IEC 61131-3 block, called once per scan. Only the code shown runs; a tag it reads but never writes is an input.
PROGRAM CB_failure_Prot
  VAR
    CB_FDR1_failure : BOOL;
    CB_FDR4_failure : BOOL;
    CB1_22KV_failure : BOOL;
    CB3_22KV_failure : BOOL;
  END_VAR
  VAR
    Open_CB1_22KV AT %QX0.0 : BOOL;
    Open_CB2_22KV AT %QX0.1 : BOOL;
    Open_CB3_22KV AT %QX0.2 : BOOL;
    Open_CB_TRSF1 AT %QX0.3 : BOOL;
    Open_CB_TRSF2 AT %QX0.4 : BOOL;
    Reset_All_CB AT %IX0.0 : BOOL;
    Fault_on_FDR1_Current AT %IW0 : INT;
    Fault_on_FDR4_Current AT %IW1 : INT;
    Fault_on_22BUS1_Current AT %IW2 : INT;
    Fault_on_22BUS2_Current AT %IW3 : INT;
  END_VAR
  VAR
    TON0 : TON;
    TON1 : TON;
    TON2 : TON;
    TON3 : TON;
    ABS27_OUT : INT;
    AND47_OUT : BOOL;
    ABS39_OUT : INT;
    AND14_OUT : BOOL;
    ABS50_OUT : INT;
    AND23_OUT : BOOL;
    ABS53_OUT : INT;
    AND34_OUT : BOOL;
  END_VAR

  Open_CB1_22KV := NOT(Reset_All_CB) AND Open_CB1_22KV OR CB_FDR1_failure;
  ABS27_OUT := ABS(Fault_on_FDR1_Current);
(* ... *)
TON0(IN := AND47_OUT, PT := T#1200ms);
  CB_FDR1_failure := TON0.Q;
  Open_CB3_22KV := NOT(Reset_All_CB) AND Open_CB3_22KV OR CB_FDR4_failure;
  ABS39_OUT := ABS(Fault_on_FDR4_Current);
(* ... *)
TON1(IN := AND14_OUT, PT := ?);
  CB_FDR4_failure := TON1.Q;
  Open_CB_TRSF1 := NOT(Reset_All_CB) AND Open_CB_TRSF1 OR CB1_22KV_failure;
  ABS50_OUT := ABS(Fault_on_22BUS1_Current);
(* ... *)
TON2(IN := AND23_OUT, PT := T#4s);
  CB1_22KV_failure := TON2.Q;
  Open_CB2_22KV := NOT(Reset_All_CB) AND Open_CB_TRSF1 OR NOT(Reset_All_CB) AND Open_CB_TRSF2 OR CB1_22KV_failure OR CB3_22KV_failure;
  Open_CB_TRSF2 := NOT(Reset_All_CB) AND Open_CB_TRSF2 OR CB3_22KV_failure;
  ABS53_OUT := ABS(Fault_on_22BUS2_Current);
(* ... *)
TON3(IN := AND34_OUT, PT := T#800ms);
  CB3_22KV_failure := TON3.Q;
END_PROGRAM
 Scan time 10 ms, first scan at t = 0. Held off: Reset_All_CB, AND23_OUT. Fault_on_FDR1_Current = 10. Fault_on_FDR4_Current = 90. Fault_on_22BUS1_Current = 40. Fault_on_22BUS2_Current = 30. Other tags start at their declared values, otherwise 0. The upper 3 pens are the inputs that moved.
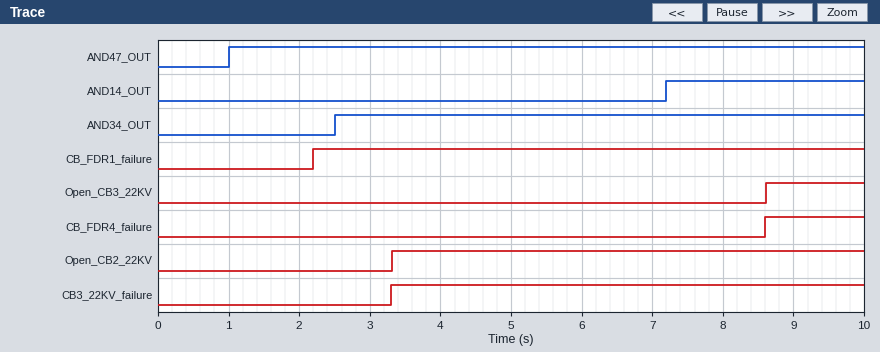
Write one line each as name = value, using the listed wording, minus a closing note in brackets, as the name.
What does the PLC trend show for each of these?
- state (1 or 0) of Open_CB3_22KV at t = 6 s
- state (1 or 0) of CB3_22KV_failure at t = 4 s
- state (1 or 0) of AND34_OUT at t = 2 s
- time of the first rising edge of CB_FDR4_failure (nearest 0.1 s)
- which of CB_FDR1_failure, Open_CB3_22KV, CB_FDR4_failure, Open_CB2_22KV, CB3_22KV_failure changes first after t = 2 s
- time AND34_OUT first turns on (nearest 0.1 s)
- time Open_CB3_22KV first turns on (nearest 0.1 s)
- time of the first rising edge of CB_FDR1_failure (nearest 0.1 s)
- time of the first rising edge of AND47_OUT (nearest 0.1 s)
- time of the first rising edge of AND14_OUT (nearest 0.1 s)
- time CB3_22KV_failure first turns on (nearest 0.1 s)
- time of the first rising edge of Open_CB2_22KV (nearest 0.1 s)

state (1 or 0) of Open_CB3_22KV at t = 6 s = 0
state (1 or 0) of CB3_22KV_failure at t = 4 s = 1
state (1 or 0) of AND34_OUT at t = 2 s = 0
time of the first rising edge of CB_FDR4_failure = 8.6 s
which of CB_FDR1_failure, Open_CB3_22KV, CB_FDR4_failure, Open_CB2_22KV, CB3_22KV_failure changes first after t = 2 s = CB_FDR1_failure
time AND34_OUT first turns on = 2.5 s
time Open_CB3_22KV first turns on = 8.6 s
time of the first rising edge of CB_FDR1_failure = 2.2 s
time of the first rising edge of AND47_OUT = 1.0 s
time of the first rising edge of AND14_OUT = 7.2 s
time CB3_22KV_failure first turns on = 3.3 s
time of the first rising edge of Open_CB2_22KV = 3.3 s
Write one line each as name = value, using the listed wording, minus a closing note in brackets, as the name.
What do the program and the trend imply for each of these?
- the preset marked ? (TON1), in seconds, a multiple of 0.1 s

the preset marked ? (TON1), in seconds, a multiple of 0.1 s = 1.4 s
